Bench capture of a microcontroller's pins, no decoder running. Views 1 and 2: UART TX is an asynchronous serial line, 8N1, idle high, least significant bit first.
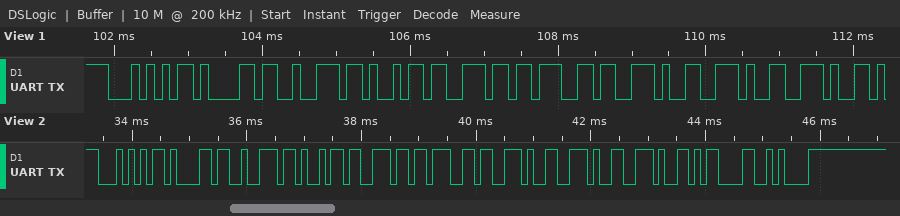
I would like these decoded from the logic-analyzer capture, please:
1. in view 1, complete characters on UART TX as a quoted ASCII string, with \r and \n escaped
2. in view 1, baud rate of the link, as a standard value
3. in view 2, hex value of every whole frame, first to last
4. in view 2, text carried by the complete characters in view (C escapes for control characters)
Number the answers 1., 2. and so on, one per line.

1. "Taring..."
2. 9600 baud
3. 0x54 0x61 0x72 0x69 0x6E 0x67 0x2E 0x2E 0x2E 0x0D 0x0A
4. "Taring...\r\n"
